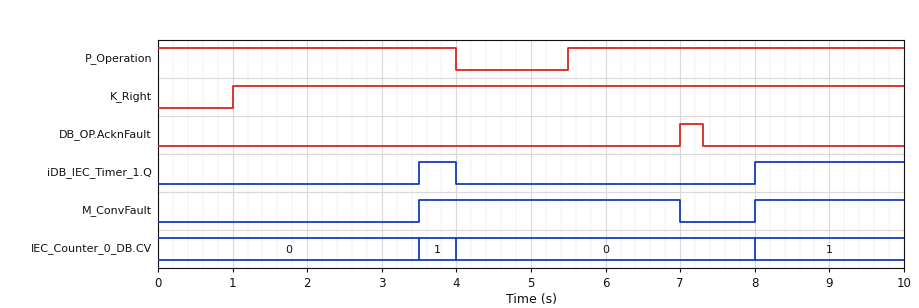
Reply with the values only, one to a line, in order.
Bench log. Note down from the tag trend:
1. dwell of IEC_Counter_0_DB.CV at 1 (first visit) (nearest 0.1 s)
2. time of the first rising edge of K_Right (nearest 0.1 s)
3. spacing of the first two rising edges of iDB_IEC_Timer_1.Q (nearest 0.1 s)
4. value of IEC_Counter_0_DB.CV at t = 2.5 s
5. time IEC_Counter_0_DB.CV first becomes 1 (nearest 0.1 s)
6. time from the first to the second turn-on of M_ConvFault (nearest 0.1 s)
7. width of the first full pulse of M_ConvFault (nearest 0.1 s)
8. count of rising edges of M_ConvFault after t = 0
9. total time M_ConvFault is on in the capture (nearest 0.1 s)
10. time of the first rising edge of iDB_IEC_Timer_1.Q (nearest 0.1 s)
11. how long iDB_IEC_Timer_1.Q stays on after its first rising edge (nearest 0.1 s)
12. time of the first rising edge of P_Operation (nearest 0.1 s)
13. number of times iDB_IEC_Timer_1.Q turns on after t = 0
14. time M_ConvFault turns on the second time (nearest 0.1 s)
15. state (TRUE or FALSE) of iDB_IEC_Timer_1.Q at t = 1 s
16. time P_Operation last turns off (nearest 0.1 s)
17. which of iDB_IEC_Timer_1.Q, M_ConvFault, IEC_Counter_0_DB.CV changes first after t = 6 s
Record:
0.5 s
1.0 s
4.5 s
0
3.5 s
4.5 s
3.5 s
2
5.5 s
3.5 s
0.5 s
5.5 s
2
8.0 s
FALSE
4.0 s
M_ConvFault
